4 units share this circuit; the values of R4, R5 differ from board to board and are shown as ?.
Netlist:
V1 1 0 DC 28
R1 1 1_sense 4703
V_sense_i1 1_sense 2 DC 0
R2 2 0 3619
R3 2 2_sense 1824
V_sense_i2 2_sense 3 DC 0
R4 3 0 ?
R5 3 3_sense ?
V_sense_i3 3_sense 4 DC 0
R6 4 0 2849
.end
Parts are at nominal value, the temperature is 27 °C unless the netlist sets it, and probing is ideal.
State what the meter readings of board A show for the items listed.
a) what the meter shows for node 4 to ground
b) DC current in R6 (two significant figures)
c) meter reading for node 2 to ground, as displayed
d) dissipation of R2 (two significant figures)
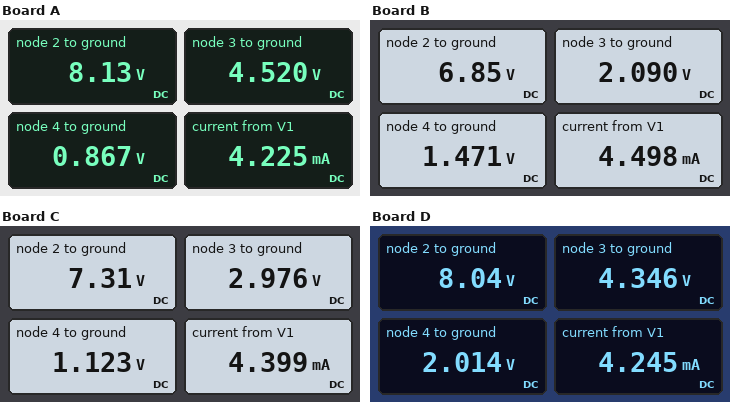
0.867 V
300 µA
8.13 V
18 mW
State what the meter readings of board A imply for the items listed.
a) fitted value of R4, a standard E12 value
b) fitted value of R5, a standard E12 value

2.7 kΩ
12 kΩ
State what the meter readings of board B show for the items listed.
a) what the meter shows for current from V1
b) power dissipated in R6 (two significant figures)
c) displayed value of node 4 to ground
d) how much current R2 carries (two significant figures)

4.498 mA
760 µW
1.471 V
1.9 mA
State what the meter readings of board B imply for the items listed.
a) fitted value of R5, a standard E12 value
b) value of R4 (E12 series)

1.2 kΩ
1 kΩ
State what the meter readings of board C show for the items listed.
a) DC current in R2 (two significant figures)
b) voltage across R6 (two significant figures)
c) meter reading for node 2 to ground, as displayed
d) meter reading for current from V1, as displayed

2.0 mA
1.1 V
7.31 V
4.399 mA
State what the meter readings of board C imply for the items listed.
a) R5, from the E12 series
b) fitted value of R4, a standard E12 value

4.7 kΩ
1.5 kΩ
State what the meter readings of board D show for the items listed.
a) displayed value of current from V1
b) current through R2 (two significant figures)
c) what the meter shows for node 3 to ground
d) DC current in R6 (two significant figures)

4.245 mA
2.2 mA
4.346 V
710 µA
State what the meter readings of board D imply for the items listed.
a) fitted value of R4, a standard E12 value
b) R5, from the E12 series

3.3 kΩ
3.3 kΩ
